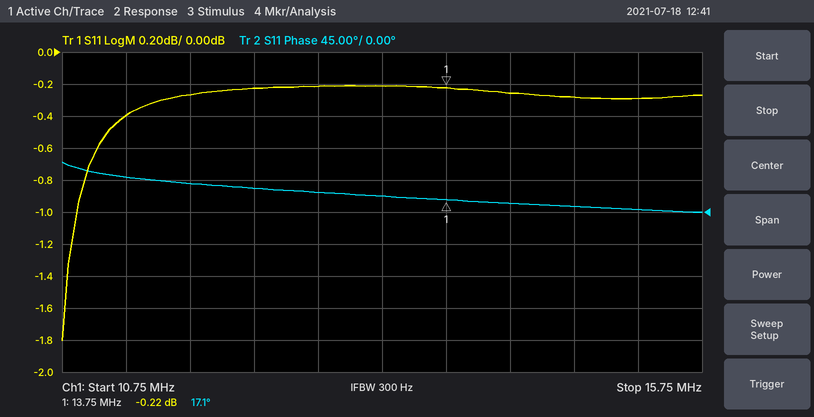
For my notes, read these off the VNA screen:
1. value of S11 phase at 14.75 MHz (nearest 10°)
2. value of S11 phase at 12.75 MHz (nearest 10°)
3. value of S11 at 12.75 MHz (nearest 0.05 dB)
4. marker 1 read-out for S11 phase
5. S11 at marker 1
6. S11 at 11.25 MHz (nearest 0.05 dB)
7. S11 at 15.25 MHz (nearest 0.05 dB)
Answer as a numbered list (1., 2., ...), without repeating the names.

1. 10°
2. 30°
3. -0.20 dB
4. 17.1°
5. -0.22 dB
6. -0.40 dB
7. -0.30 dB
